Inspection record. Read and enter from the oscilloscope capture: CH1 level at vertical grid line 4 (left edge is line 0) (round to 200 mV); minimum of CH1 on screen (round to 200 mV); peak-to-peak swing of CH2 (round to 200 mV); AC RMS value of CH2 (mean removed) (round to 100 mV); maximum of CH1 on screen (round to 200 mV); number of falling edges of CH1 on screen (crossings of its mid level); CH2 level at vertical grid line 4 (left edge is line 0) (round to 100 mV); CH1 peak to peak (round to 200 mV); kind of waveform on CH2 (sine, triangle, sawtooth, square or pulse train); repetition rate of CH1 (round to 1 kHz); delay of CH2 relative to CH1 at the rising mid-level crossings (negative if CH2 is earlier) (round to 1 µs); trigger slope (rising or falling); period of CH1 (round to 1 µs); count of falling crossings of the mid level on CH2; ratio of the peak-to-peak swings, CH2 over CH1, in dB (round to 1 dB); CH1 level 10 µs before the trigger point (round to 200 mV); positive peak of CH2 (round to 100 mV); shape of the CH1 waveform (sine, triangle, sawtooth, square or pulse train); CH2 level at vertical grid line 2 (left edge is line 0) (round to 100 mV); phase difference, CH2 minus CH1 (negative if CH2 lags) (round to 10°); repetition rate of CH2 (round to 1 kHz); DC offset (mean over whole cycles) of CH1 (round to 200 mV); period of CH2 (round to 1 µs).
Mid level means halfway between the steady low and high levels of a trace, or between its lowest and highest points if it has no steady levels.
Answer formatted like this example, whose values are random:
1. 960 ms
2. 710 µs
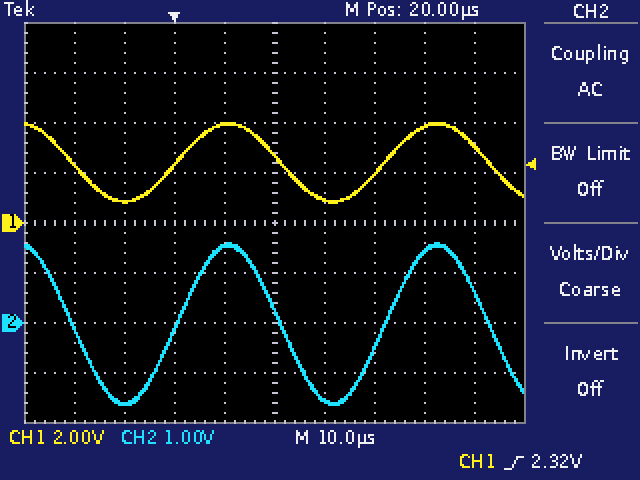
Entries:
1. 4.0 V
2. 800 mV
3. 3.2 V
4. 1.1 V
5. 4.0 V
6. 3
7. 1.5 V
8. 3.2 V
9. sine
10. 24 kHz
11. 0 µs
12. rising
13. 42 µs
14. 3
15. 0 dB
16. 800 mV
17. 1.6 V
18. sine
19. -1.6 V
20. 0°
21. 24 kHz
22. 2.4 V
23. 42 µs
